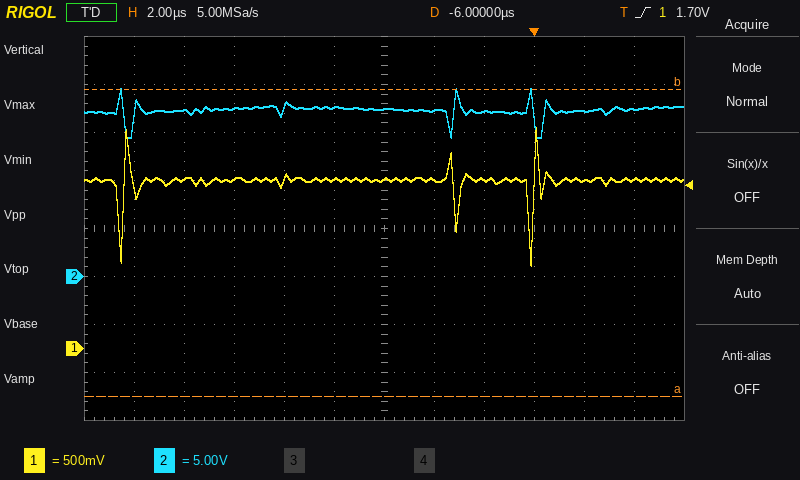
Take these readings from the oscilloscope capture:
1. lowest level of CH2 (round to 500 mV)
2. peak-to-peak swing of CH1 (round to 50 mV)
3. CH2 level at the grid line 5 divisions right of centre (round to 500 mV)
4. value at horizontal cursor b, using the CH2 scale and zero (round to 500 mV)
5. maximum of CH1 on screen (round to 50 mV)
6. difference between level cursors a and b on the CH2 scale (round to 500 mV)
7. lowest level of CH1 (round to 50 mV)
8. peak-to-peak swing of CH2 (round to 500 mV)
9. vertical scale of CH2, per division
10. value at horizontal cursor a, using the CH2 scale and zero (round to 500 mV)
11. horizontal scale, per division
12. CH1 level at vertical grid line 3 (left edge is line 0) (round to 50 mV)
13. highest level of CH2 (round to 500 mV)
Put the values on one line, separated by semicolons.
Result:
14.5 V; 1.45 V; 17.5 V; 19.5 V; 2.30 V; 32.0 V; 850 mV; 5.0 V; 5 V; -12.5 V; 2 µs; 1.75 V; 19.5 V
